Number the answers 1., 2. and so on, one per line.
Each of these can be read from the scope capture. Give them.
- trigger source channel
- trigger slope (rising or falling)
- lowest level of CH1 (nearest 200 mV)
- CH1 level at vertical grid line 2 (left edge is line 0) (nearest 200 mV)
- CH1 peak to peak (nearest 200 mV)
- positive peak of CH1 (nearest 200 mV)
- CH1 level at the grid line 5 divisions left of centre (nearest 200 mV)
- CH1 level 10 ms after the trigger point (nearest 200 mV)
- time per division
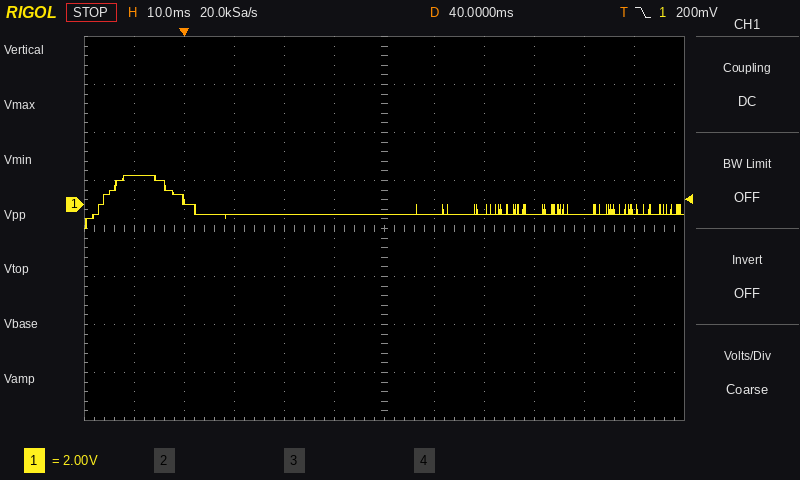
1. CH1
2. falling
3. -1.0 V
4. 200 mV
5. 2.2 V
6. 1.2 V
7. 1.2 V
8. -400 mV
9. 10 ms
